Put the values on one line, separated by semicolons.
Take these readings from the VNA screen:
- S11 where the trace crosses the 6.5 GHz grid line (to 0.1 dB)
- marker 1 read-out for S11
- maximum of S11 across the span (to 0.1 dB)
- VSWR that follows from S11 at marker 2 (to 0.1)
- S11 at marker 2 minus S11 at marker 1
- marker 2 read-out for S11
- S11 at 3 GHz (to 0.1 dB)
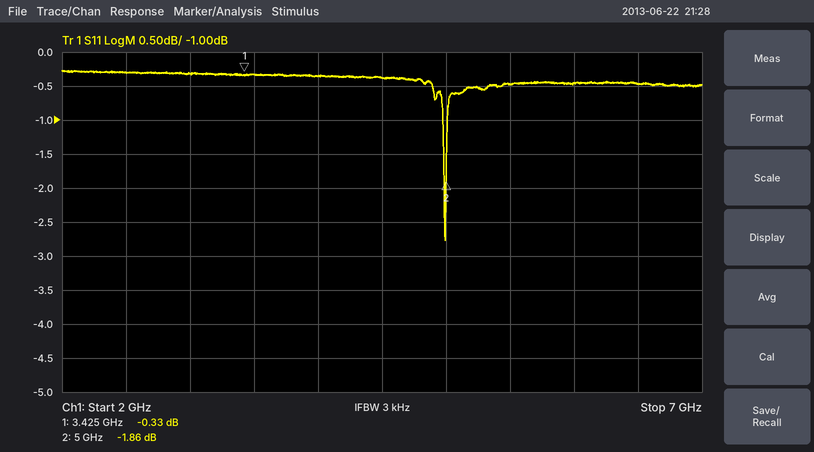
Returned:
-0.5 dB; -0.33 dB; -0.3 dB; 9.4; -1.53 dB; -1.86 dB; -0.3 dB
